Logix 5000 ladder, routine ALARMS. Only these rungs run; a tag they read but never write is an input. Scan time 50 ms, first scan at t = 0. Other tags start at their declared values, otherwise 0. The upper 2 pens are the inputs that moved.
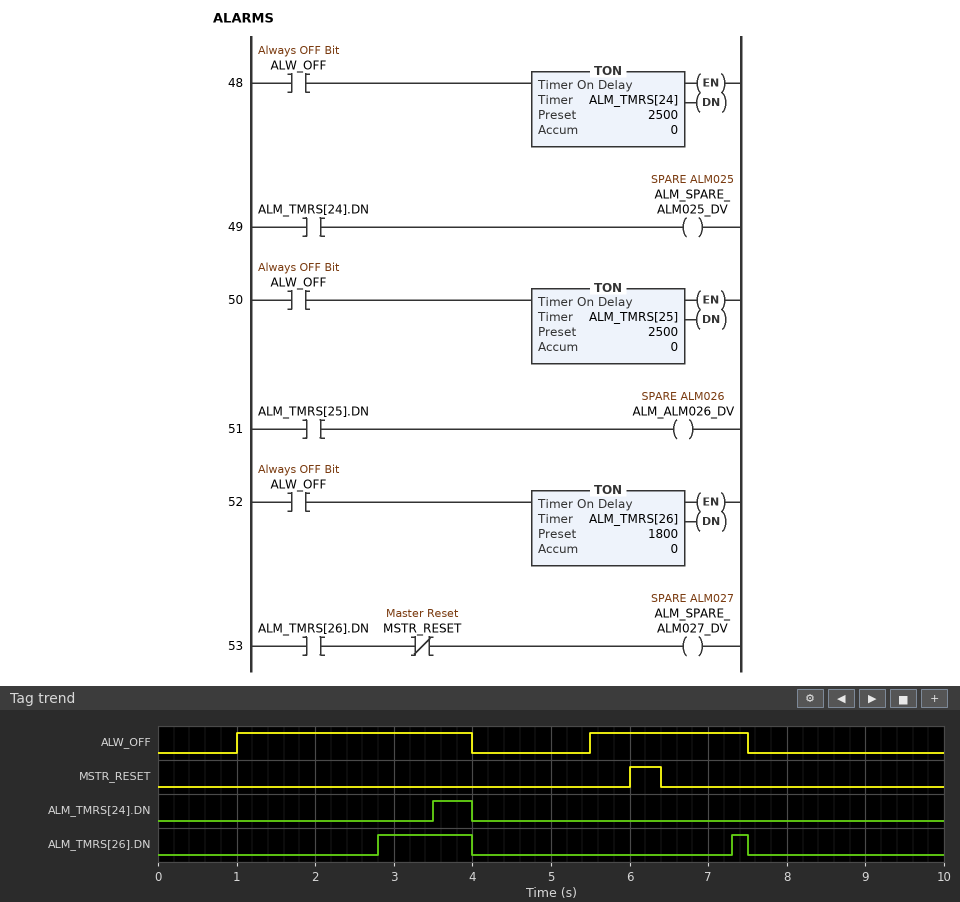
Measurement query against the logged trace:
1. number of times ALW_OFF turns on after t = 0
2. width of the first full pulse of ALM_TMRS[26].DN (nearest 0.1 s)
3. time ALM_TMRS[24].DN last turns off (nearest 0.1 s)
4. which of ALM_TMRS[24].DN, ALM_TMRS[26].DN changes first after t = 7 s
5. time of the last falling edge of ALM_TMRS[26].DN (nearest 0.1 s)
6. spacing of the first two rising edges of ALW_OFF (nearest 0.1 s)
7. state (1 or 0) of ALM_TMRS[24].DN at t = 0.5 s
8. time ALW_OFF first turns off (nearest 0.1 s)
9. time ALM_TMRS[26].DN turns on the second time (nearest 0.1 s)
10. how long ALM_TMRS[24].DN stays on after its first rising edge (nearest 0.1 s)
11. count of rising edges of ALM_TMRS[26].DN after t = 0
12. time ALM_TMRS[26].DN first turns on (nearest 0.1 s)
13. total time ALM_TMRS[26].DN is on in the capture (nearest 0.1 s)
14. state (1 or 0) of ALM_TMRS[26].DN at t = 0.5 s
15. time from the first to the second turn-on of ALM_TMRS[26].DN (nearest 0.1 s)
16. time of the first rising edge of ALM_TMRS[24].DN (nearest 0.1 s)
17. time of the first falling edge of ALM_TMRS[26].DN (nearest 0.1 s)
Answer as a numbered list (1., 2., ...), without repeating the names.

1. 2
2. 1.2 s
3. 4.0 s
4. ALM_TMRS[26].DN
5. 7.5 s
6. 4.5 s
7. 0
8. 4.0 s
9. 7.3 s
10. 0.5 s
11. 2
12. 2.8 s
13. 1.4 s
14. 0
15. 4.5 s
16. 3.5 s
17. 4.0 s
